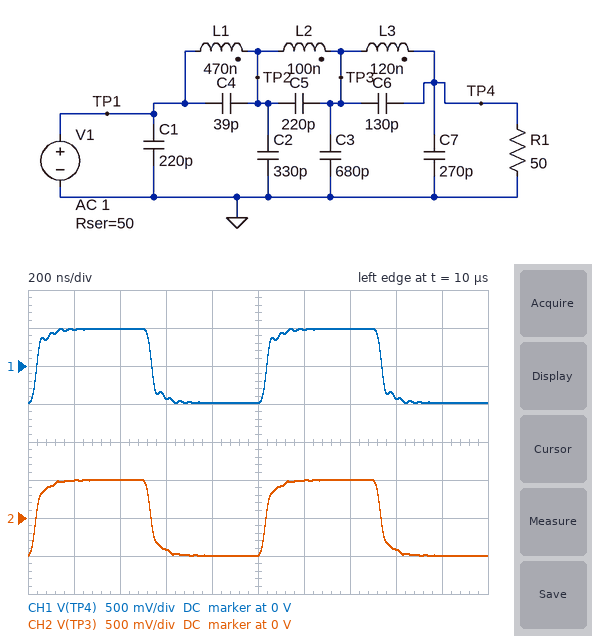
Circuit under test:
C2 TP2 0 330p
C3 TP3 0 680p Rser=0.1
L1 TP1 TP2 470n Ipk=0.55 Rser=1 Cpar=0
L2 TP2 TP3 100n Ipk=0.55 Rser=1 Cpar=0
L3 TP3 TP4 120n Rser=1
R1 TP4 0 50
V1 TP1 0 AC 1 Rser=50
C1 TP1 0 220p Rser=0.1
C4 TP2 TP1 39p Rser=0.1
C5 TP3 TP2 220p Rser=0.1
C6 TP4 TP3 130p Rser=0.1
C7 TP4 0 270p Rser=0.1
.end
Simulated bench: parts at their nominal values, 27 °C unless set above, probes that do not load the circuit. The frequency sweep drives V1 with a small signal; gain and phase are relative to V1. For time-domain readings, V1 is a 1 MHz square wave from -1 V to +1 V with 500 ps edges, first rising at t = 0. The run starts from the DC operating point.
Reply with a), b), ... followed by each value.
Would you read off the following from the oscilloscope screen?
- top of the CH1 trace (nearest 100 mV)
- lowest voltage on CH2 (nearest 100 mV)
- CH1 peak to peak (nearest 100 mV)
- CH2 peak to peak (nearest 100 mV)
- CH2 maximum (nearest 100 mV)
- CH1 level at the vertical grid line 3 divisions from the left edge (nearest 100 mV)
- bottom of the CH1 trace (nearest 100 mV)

a) 500 mV
b) -500 mV
c) 1.0 V
d) 1.0 V
e) 500 mV
f) -400 mV
g) -500 mV
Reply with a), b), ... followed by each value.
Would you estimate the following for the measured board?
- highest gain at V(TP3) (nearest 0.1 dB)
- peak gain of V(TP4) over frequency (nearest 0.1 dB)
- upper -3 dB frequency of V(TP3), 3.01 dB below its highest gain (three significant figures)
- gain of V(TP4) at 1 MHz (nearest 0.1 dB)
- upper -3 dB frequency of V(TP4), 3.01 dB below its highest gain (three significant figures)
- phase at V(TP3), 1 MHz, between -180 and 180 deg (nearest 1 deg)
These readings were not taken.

a) -6.1 dB
b) -6.3 dB
c) 5.53 MHz
d) -6.4 dB
e) 6.17 MHz
f) -15 deg
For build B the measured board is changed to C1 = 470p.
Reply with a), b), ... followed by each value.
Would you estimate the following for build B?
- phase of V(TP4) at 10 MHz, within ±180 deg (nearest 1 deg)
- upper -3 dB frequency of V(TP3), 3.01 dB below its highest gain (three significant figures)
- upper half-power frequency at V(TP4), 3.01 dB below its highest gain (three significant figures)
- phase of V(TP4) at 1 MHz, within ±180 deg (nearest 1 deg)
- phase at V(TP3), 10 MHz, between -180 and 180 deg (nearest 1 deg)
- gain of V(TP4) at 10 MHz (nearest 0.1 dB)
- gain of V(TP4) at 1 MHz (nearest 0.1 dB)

a) -144 deg
b) 5.30 MHz
c) 11.2 MHz
d) -18 deg
e) -132 deg
f) -8.5 dB
g) -6.5 dB
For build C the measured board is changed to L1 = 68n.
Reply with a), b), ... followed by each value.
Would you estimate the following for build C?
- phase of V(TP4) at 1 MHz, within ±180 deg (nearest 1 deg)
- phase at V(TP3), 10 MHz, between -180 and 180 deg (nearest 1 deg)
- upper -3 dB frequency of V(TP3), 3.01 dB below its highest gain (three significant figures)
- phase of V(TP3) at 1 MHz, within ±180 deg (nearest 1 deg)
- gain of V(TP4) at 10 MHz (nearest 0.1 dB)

a) -15 deg
b) -75 deg
c) 4.59 MHz
d) -14 deg
e) -11.8 dB
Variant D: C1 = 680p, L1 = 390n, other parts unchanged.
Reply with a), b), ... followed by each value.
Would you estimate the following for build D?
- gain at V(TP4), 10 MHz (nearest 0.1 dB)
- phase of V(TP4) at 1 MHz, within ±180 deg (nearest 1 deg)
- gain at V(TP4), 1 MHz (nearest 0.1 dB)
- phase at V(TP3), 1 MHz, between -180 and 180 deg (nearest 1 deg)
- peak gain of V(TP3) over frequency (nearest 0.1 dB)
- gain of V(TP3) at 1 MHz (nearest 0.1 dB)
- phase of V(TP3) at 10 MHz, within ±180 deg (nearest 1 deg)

a) -7.9 dB
b) -20 deg
c) -6.6 dB
d) -19 deg
e) -6.1 dB
f) -6.4 dB
g) -136 deg
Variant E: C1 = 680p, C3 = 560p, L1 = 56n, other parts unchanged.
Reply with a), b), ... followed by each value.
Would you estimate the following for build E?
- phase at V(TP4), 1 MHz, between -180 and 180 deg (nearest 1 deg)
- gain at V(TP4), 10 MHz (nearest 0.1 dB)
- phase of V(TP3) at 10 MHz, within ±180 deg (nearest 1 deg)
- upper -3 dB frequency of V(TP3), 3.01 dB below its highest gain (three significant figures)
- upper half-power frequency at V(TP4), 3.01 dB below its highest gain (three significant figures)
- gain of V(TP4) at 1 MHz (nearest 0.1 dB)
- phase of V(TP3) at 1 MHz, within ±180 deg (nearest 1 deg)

a) -18 deg
b) -12.5 dB
c) -81 deg
d) 3.72 MHz
e) 3.85 MHz
f) -6.6 dB
g) -17 deg
